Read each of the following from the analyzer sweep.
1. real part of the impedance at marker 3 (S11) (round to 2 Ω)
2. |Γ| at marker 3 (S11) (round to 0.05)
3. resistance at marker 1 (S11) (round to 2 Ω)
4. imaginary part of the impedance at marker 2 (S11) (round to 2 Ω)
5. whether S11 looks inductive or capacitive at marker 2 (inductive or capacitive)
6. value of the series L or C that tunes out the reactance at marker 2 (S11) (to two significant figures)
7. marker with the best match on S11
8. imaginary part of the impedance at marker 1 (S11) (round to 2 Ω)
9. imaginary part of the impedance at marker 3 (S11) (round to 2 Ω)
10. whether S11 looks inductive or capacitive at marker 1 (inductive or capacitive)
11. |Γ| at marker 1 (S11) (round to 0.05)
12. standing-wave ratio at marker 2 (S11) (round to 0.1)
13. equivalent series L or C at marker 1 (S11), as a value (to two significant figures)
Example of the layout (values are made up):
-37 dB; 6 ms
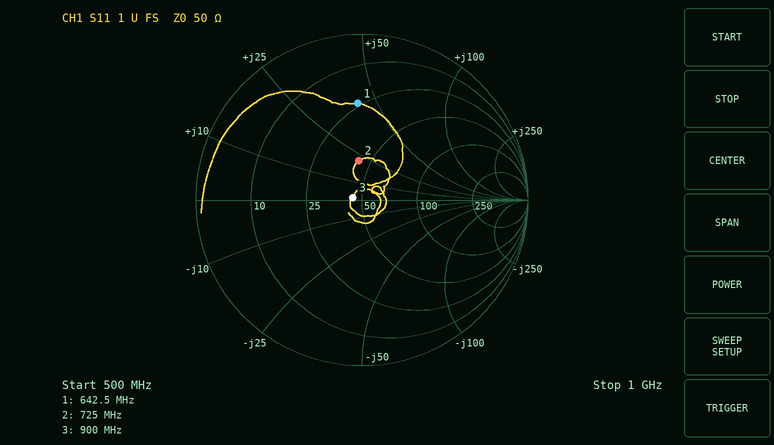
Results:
44 Ω; 0.05; 24 Ω; +22 Ω; inductive; 10 pF; marker 3; +42 Ω; +2 Ω; inductive; 0.60; 1.6; 10 nH
